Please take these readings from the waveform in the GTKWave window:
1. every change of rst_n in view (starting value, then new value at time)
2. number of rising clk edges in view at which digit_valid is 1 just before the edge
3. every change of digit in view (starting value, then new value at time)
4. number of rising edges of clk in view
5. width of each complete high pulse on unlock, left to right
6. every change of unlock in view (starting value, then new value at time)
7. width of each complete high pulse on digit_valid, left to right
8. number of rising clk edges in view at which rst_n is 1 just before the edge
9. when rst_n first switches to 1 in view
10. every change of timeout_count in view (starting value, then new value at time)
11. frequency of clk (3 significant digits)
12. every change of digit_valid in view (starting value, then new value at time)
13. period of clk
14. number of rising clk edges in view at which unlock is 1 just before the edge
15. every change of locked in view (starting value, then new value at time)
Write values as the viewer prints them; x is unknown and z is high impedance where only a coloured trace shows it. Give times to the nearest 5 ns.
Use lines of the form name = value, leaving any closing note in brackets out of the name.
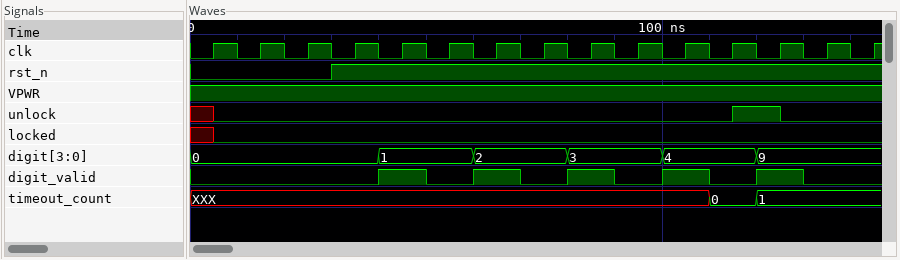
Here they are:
every change of rst_n in view = 0, 1 at 30 ns
number of rising clk edges in view at which digit_valid is 1 just before the edge = 5
every change of digit in view = 0, 1 at 40 ns, 2 at 60 ns, 3 at 80 ns, 4 at 100 ns, 9 at 120 ns
number of rising edges of clk in view = 15
width of each complete high pulse on unlock, left to right = 10 ns
every change of unlock in view = x, 0 at 5 ns, 1 at 115 ns, 0 at 125 ns
width of each complete high pulse on digit_valid, left to right = 10 ns, 10 ns, 10 ns, 10 ns, 10 ns
number of rising clk edges in view at which rst_n is 1 just before the edge = 12
when rst_n first switches to 1 in view = 30 ns
every change of timeout_count in view = XXX, 0 at 110 ns, 1 at 120 ns
frequency of clk = 100 MHz
every change of digit_valid in view = 0, 1 at 40 ns, 0 at 50 ns, 1 at 60 ns, 0 at 70 ns, 1 at 80 ns, 0 at 90 ns, 1 at 100 ns, 0 at 110 ns, 1 at 120 ns, 0 at 130 ns
period of clk = 10 ns
number of rising clk edges in view at which unlock is 1 just before the edge = 1
every change of locked in view = x, 0 at 5 ns
